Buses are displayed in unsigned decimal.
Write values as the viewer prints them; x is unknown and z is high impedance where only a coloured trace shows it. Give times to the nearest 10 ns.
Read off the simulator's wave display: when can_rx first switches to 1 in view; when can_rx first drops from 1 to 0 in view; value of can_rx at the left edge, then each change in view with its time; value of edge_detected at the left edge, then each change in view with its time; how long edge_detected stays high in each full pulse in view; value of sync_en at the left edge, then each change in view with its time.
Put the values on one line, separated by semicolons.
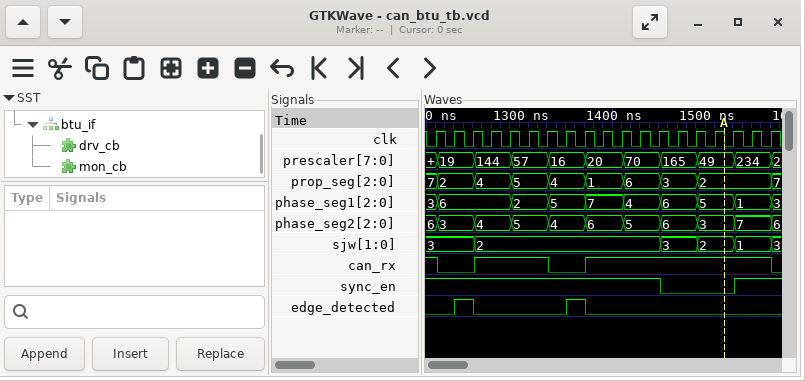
1250 ns; 1210 ns; 1, 0 at 1210 ns, 1 at 1250 ns, 0 at 1330 ns, 1 at 1370 ns, 0 at 1570 ns; 0, 1 at 1230 ns, 0 at 1250 ns, 1 at 1350 ns, 0 at 1370 ns; 20 ns, 20 ns; 1, 0 at 1450 ns, 1 at 1530 ns
